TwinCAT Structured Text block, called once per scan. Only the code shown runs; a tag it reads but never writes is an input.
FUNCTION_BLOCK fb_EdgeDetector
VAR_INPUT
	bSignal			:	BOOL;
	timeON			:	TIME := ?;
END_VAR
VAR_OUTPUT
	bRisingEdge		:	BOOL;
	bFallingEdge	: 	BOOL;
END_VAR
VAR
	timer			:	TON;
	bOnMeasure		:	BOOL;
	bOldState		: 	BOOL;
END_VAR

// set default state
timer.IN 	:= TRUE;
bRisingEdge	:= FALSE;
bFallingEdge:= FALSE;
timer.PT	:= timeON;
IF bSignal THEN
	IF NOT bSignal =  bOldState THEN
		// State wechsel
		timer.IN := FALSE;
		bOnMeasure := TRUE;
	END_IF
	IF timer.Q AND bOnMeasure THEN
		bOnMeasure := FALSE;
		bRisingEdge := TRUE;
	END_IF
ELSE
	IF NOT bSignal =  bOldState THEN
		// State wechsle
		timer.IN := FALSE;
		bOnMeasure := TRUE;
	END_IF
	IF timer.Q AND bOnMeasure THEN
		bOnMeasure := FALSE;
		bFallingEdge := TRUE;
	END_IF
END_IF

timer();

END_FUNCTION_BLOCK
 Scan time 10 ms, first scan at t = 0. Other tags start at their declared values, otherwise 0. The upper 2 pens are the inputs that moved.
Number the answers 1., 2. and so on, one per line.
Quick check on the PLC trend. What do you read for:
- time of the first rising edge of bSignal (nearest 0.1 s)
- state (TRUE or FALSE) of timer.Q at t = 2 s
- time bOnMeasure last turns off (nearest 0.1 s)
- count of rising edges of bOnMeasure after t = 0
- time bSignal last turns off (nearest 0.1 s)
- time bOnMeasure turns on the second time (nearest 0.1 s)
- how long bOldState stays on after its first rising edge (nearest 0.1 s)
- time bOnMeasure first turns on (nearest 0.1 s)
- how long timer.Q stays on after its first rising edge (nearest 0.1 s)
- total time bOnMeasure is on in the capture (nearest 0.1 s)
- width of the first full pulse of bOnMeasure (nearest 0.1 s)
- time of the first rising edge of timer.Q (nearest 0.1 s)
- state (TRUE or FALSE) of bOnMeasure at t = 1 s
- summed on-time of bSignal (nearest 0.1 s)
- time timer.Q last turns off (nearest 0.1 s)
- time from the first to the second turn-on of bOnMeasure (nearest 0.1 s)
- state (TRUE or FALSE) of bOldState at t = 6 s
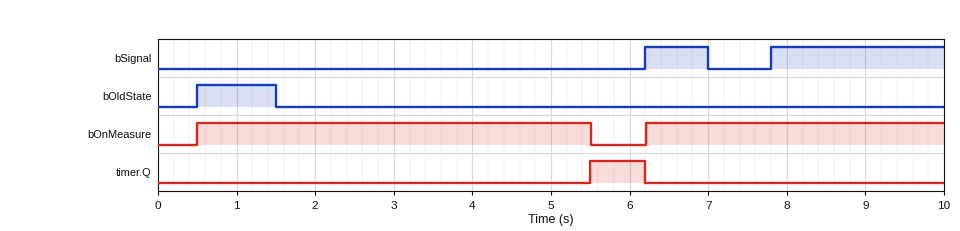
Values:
1. 6.2 s
2. FALSE
3. 5.5 s
4. 2
5. 7.0 s
6. 6.2 s
7. 1.0 s
8. 0.5 s
9. 0.7 s
10. 8.8 s
11. 5.0 s
12. 5.5 s
13. TRUE
14. 3.0 s
15. 6.2 s
16. 5.7 s
17. FALSE
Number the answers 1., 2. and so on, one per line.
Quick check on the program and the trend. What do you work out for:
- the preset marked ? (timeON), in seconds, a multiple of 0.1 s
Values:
1. 4.0 s
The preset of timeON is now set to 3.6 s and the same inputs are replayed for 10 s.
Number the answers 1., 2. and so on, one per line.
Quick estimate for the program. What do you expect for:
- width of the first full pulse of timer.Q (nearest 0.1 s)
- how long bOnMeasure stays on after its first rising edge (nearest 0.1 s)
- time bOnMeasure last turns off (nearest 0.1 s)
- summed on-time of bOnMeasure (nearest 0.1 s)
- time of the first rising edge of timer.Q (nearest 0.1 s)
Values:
1. 1.1 s
2. 4.6 s
3. 5.1 s
4. 8.4 s
5. 5.1 s
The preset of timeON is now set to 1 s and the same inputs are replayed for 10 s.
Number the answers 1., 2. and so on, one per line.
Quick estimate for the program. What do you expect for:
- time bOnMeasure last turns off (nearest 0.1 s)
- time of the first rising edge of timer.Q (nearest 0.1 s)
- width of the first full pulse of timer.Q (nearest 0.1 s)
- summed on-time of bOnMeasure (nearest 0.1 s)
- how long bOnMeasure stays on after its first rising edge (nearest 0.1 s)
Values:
1. 2.5 s
2. 2.5 s
3. 3.7 s
4. 5.8 s
5. 2.0 s
